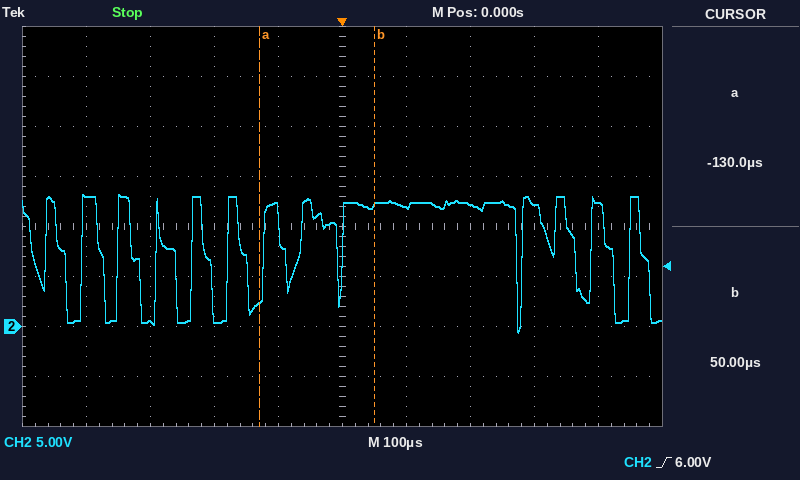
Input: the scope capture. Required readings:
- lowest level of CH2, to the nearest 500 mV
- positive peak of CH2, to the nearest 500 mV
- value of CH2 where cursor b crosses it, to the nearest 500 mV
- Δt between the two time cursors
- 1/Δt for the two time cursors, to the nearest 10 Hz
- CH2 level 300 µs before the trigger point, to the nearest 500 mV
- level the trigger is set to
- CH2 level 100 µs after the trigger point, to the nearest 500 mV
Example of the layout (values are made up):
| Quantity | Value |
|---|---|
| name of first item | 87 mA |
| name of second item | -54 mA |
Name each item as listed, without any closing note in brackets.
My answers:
| Quantity | Value |
|---|---|
| lowest level of CH2, to the nearest 500 mV | -500 mV |
| positive peak of CH2, to the nearest 500 mV | 13.0 V |
| value of CH2 where cursor b crosses it, to the nearest 500 mV | 12.0 V |
| Δt between the two time cursors | 180 µs |
| 1/Δt for the two time cursors, to the nearest 10 Hz | 5.56 kHz |
| CH2 level 300 µs before the trigger point, to the nearest 500 mV | 500 mV |
| level the trigger is set to | 6.00 V |
| CH2 level 100 µs after the trigger point, to the nearest 500 mV | 12.0 V |
